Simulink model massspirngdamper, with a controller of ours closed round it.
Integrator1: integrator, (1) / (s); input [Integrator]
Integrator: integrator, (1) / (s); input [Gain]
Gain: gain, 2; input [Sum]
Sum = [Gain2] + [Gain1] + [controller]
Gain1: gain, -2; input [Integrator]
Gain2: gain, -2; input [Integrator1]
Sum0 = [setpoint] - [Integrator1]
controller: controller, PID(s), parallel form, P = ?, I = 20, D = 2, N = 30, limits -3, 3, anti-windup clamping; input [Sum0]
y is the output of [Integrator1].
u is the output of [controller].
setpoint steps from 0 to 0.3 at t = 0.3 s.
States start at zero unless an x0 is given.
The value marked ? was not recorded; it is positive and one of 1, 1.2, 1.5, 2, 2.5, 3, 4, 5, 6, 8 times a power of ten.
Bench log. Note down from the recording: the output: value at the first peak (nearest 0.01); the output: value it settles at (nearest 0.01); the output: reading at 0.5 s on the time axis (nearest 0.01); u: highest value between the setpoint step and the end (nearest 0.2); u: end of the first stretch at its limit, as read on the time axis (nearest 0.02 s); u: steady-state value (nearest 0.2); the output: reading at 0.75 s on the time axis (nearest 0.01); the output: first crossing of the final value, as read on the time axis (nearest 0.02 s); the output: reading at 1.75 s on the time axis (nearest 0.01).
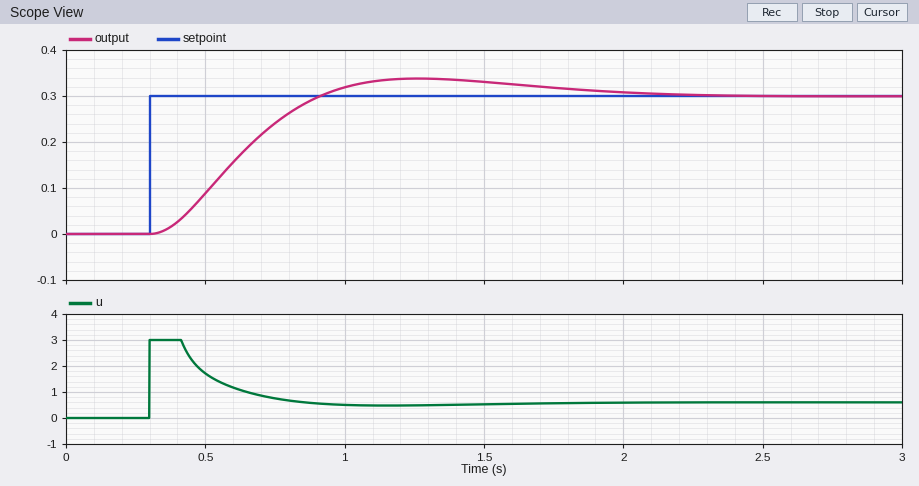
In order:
0.34
0.30
0.09
3.0
0.42 s
0.6
0.24
0.92 s
0.32
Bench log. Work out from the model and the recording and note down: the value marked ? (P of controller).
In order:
12
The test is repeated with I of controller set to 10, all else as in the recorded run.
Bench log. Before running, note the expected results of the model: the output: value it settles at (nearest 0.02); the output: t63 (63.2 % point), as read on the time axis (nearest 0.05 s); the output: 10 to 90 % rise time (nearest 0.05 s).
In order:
0.30
0.65 s
0.50 s
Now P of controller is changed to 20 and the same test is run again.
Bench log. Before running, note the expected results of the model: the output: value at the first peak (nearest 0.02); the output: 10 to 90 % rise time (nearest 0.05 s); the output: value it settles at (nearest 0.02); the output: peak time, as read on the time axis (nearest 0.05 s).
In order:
0.32
0.35 s
0.30
1.00 s
